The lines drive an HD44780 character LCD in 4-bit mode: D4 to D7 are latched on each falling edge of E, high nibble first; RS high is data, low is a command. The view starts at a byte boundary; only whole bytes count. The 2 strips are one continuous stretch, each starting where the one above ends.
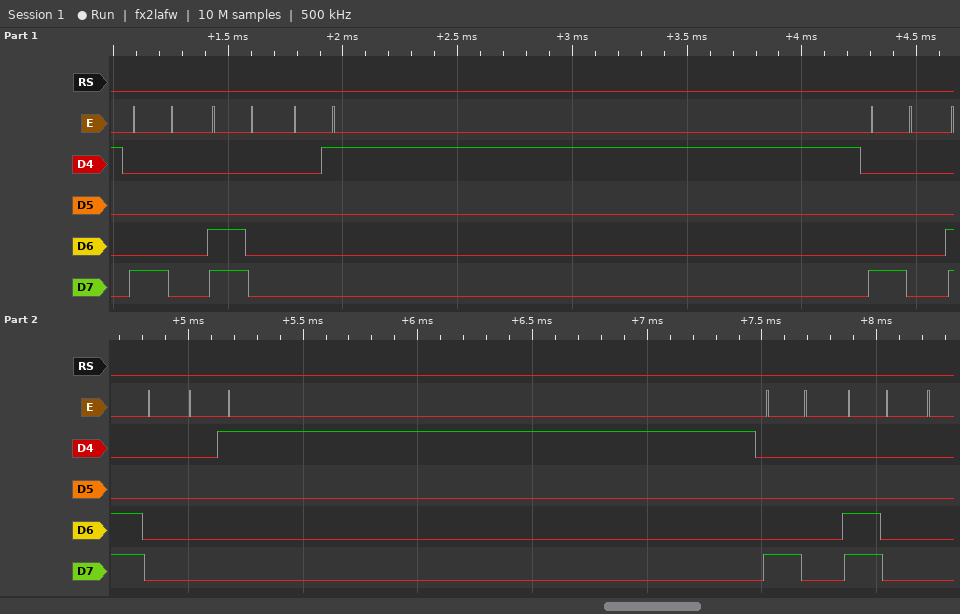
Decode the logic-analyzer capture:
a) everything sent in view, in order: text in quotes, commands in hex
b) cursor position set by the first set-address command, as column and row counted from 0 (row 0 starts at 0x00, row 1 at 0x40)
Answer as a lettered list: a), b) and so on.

a) 0x80 0xC0 0x01 0x80 0xC0 0x01 0x80 0xC0
b) column 0, row 0
